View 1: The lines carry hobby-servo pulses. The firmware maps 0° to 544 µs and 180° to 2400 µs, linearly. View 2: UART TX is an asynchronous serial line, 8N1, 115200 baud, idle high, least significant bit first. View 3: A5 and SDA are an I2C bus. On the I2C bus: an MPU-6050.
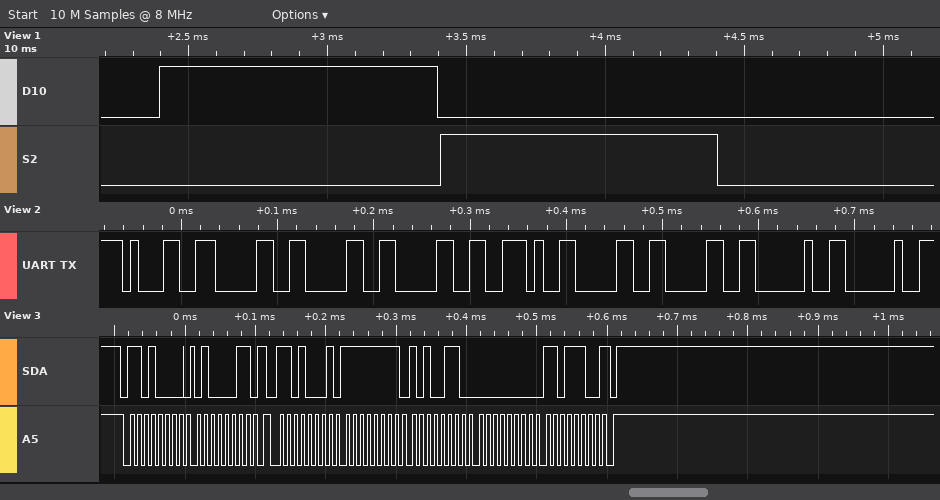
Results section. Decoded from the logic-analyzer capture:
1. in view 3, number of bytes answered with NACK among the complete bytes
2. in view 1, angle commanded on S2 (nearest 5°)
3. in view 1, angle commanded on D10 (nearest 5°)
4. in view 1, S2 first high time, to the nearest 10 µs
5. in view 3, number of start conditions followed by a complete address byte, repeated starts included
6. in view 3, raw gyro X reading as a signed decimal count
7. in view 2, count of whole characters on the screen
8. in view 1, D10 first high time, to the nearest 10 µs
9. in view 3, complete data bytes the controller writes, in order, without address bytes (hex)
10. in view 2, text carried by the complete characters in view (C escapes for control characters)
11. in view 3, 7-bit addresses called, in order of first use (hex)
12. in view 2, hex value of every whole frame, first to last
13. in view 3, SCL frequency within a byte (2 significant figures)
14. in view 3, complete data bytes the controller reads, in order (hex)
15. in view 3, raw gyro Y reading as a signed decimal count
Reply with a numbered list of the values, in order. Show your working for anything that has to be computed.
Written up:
1. 1
2. 45°
3. 45°
4. 1000 µs
5. 2
6. 0xFFA6 = -90
7. 9
8. 1000 µs
9. 43
10. "1000.00  "
11. 0x68
12. 31 30 30 30 2E 30 30 20 20
13. 100 kHz
14. FF A6 00 DC
15. 0x00DC = 220
